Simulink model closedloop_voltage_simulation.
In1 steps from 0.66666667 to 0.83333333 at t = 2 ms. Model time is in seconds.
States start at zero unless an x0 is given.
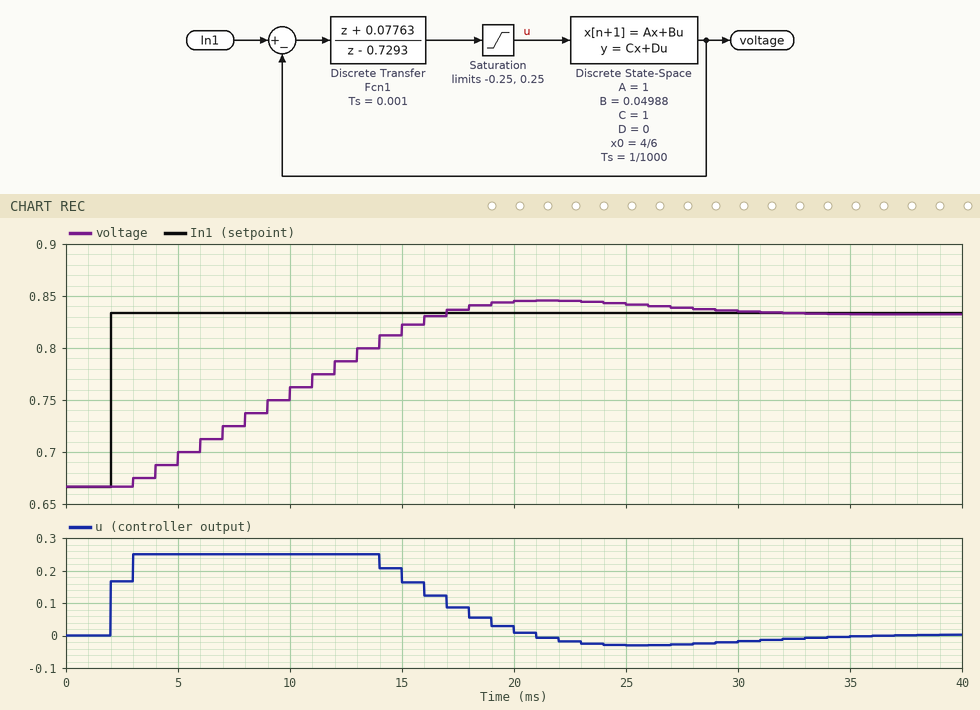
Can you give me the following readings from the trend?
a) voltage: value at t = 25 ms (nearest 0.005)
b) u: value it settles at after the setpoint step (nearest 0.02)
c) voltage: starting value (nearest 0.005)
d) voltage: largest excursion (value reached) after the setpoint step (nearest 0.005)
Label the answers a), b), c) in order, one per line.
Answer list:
a) 0.840
b) 0.00
c) 0.665
d) 0.845
